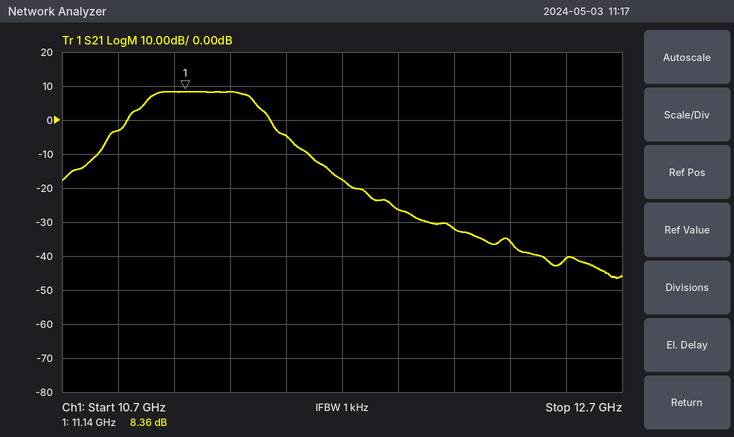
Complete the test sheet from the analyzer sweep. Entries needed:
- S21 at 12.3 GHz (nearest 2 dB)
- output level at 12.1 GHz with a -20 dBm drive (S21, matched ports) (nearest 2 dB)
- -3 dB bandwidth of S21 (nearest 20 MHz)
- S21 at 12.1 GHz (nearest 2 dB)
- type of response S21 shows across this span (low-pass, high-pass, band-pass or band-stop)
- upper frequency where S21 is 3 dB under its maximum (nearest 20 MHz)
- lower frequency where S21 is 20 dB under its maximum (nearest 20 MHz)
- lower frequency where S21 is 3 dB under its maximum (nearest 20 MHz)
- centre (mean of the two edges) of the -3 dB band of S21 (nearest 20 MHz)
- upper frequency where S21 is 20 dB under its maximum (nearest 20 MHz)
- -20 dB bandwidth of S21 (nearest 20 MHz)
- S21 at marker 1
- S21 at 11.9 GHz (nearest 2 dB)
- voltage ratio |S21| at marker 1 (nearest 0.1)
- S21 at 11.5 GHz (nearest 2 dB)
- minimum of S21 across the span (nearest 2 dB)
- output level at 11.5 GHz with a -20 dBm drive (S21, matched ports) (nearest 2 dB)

-36 dB
-52 dBm
380 MHz
-32 dB
band-pass
11.38 GHz
10.80 GHz
11.00 GHz
11.20 GHz
11.60 GHz
800 MHz
8.36 dB
-26 dB
2.6
-4 dB
-46 dB
-24 dBm
